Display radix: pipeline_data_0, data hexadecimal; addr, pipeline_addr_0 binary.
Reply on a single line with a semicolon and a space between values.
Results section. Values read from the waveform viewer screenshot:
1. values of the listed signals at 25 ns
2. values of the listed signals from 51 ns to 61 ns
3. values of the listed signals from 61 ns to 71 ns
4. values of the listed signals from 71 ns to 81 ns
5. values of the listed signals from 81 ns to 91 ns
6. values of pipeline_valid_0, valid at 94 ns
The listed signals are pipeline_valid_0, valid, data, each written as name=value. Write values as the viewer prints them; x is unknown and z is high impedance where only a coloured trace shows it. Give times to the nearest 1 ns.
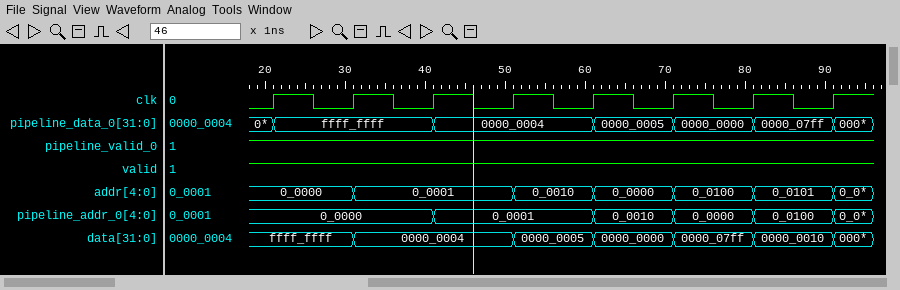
pipeline_valid_0=1, valid=1, data=ffff_ffff; pipeline_valid_0=1, valid=1, data=0000_0005; pipeline_valid_0=1, valid=1, data=0000_0000; pipeline_valid_0=1, valid=1, data=0000_07ff; pipeline_valid_0=1, valid=1, data=0000_0010; pipeline_valid_0=1, valid=1
